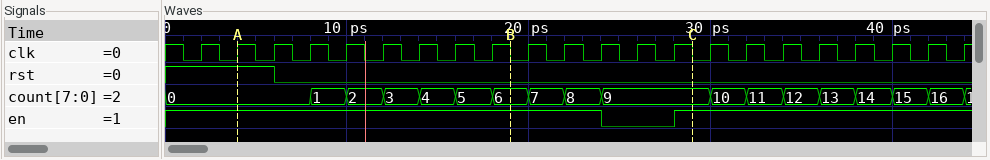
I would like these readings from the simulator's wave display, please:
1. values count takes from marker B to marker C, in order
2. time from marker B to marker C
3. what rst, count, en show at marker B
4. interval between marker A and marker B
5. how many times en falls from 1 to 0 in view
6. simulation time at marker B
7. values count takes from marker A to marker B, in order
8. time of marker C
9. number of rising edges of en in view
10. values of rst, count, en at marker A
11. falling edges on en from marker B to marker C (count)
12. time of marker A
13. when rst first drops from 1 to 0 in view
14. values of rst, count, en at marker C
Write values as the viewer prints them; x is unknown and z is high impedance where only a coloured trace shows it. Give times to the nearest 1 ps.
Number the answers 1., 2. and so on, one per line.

1. 6, 7, 8, 9
2. 10 ps
3. rst=0, count=6, en=1
4. 15 ps
5. 1
6. 19 ps
7. 0, 1, 2, 3, 4, 5, 6
8. 29 ps
9. 1
10. rst=1, count=0, en=1
11. 1
12. 4 ps
13. 6 ps
14. rst=0, count=9, en=1
